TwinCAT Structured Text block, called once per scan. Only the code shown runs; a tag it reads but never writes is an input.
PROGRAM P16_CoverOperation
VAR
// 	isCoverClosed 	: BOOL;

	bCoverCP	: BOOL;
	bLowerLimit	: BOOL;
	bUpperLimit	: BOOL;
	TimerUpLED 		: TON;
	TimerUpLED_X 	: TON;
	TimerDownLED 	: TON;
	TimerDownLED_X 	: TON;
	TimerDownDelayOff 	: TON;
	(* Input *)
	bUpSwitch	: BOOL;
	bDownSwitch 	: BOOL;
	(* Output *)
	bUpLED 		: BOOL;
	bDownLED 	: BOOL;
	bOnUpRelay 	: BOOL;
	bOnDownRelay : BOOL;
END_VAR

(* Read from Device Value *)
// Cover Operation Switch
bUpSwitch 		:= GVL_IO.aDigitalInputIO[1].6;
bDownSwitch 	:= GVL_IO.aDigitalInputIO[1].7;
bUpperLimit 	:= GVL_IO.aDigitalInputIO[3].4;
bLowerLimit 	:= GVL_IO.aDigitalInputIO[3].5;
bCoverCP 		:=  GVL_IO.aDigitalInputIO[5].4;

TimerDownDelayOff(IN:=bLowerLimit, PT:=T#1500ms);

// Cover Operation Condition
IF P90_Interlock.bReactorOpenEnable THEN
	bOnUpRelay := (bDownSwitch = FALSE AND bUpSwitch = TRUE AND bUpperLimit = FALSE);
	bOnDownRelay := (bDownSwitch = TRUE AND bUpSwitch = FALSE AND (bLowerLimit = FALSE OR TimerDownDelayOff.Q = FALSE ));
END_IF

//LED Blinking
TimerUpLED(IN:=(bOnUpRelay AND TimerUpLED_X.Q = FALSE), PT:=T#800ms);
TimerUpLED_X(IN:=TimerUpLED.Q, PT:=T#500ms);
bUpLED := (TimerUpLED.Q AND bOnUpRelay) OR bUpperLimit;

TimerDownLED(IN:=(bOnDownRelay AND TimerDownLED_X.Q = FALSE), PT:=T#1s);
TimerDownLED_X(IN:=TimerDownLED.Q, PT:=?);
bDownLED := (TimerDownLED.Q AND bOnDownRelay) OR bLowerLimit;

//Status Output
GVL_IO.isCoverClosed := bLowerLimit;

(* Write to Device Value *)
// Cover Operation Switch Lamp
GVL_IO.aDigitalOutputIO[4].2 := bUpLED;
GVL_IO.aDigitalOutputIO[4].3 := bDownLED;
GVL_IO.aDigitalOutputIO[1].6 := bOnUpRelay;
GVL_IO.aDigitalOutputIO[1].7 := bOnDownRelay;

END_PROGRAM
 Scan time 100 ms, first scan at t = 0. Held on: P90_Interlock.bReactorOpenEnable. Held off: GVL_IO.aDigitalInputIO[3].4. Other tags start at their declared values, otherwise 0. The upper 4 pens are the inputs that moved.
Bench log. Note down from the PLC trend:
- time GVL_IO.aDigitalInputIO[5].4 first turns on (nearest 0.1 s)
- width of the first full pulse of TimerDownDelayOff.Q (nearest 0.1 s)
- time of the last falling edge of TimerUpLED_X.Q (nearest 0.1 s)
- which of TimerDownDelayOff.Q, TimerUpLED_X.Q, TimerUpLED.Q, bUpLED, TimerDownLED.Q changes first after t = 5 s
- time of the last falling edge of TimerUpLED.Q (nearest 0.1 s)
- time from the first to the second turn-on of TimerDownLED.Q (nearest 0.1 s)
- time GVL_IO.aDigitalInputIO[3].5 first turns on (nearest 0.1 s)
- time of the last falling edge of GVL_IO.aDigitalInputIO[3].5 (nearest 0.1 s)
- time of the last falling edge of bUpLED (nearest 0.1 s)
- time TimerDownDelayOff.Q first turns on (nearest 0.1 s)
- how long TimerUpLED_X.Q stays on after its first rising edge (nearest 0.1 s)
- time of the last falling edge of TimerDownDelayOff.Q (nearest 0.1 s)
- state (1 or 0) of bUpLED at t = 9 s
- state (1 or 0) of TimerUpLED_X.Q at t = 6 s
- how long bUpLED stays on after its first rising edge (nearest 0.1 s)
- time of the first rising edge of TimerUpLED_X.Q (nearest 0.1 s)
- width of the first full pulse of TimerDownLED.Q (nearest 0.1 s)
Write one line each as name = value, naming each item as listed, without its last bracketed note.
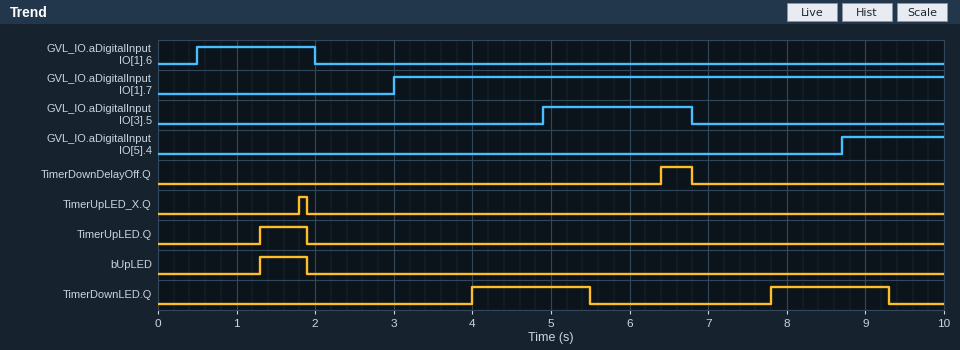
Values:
time GVL_IO.aDigitalInputIO[5].4 first turns on = 8.7 s
width of the first full pulse of TimerDownDelayOff.Q = 0.4 s
time of the last falling edge of TimerUpLED_X.Q = 1.9 s
which of TimerDownDelayOff.Q, TimerUpLED_X.Q, TimerUpLED.Q, bUpLED, TimerDownLED.Q changes first after t = 5 s = TimerDownLED.Q
time of the last falling edge of TimerUpLED.Q = 1.9 s
time from the first to the second turn-on of TimerDownLED.Q = 3.8 s
time GVL_IO.aDigitalInputIO[3].5 first turns on = 4.9 s
time of the last falling edge of GVL_IO.aDigitalInputIO[3].5 = 6.8 s
time of the last falling edge of bUpLED = 1.9 s
time TimerDownDelayOff.Q first turns on = 6.4 s
how long TimerUpLED_X.Q stays on after its first rising edge = 0.1 s
time of the last falling edge of TimerDownDelayOff.Q = 6.8 s
state (1 or 0) of bUpLED at t = 9 s = 0
state (1 or 0) of TimerUpLED_X.Q at t = 6 s = 0
how long bUpLED stays on after its first rising edge = 0.6 s
time of the first rising edge of TimerUpLED_X.Q = 1.8 s
width of the first full pulse of TimerDownLED.Q = 1.5 s
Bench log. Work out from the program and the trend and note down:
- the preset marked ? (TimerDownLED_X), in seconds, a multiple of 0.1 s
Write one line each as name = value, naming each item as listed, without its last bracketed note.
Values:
the preset marked ? (TimerDownLED_X), in seconds, a multiple of 0.1 s = 1.4 s
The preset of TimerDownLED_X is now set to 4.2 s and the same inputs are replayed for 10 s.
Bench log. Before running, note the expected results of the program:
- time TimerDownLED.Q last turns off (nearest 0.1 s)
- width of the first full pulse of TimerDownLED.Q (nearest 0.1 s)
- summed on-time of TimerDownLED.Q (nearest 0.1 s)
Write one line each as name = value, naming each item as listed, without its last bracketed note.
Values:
time TimerDownLED.Q last turns off = 6.4 s
width of the first full pulse of TimerDownLED.Q = 2.4 s
summed on-time of TimerDownLED.Q = 4.6 s
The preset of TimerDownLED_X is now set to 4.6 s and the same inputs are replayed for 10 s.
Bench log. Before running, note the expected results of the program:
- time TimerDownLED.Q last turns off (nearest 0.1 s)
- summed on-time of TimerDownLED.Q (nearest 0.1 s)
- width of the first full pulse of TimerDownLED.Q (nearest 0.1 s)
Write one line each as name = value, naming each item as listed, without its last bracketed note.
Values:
time TimerDownLED.Q last turns off = 6.4 s
summed on-time of TimerDownLED.Q = 4.6 s
width of the first full pulse of TimerDownLED.Q = 2.4 s
